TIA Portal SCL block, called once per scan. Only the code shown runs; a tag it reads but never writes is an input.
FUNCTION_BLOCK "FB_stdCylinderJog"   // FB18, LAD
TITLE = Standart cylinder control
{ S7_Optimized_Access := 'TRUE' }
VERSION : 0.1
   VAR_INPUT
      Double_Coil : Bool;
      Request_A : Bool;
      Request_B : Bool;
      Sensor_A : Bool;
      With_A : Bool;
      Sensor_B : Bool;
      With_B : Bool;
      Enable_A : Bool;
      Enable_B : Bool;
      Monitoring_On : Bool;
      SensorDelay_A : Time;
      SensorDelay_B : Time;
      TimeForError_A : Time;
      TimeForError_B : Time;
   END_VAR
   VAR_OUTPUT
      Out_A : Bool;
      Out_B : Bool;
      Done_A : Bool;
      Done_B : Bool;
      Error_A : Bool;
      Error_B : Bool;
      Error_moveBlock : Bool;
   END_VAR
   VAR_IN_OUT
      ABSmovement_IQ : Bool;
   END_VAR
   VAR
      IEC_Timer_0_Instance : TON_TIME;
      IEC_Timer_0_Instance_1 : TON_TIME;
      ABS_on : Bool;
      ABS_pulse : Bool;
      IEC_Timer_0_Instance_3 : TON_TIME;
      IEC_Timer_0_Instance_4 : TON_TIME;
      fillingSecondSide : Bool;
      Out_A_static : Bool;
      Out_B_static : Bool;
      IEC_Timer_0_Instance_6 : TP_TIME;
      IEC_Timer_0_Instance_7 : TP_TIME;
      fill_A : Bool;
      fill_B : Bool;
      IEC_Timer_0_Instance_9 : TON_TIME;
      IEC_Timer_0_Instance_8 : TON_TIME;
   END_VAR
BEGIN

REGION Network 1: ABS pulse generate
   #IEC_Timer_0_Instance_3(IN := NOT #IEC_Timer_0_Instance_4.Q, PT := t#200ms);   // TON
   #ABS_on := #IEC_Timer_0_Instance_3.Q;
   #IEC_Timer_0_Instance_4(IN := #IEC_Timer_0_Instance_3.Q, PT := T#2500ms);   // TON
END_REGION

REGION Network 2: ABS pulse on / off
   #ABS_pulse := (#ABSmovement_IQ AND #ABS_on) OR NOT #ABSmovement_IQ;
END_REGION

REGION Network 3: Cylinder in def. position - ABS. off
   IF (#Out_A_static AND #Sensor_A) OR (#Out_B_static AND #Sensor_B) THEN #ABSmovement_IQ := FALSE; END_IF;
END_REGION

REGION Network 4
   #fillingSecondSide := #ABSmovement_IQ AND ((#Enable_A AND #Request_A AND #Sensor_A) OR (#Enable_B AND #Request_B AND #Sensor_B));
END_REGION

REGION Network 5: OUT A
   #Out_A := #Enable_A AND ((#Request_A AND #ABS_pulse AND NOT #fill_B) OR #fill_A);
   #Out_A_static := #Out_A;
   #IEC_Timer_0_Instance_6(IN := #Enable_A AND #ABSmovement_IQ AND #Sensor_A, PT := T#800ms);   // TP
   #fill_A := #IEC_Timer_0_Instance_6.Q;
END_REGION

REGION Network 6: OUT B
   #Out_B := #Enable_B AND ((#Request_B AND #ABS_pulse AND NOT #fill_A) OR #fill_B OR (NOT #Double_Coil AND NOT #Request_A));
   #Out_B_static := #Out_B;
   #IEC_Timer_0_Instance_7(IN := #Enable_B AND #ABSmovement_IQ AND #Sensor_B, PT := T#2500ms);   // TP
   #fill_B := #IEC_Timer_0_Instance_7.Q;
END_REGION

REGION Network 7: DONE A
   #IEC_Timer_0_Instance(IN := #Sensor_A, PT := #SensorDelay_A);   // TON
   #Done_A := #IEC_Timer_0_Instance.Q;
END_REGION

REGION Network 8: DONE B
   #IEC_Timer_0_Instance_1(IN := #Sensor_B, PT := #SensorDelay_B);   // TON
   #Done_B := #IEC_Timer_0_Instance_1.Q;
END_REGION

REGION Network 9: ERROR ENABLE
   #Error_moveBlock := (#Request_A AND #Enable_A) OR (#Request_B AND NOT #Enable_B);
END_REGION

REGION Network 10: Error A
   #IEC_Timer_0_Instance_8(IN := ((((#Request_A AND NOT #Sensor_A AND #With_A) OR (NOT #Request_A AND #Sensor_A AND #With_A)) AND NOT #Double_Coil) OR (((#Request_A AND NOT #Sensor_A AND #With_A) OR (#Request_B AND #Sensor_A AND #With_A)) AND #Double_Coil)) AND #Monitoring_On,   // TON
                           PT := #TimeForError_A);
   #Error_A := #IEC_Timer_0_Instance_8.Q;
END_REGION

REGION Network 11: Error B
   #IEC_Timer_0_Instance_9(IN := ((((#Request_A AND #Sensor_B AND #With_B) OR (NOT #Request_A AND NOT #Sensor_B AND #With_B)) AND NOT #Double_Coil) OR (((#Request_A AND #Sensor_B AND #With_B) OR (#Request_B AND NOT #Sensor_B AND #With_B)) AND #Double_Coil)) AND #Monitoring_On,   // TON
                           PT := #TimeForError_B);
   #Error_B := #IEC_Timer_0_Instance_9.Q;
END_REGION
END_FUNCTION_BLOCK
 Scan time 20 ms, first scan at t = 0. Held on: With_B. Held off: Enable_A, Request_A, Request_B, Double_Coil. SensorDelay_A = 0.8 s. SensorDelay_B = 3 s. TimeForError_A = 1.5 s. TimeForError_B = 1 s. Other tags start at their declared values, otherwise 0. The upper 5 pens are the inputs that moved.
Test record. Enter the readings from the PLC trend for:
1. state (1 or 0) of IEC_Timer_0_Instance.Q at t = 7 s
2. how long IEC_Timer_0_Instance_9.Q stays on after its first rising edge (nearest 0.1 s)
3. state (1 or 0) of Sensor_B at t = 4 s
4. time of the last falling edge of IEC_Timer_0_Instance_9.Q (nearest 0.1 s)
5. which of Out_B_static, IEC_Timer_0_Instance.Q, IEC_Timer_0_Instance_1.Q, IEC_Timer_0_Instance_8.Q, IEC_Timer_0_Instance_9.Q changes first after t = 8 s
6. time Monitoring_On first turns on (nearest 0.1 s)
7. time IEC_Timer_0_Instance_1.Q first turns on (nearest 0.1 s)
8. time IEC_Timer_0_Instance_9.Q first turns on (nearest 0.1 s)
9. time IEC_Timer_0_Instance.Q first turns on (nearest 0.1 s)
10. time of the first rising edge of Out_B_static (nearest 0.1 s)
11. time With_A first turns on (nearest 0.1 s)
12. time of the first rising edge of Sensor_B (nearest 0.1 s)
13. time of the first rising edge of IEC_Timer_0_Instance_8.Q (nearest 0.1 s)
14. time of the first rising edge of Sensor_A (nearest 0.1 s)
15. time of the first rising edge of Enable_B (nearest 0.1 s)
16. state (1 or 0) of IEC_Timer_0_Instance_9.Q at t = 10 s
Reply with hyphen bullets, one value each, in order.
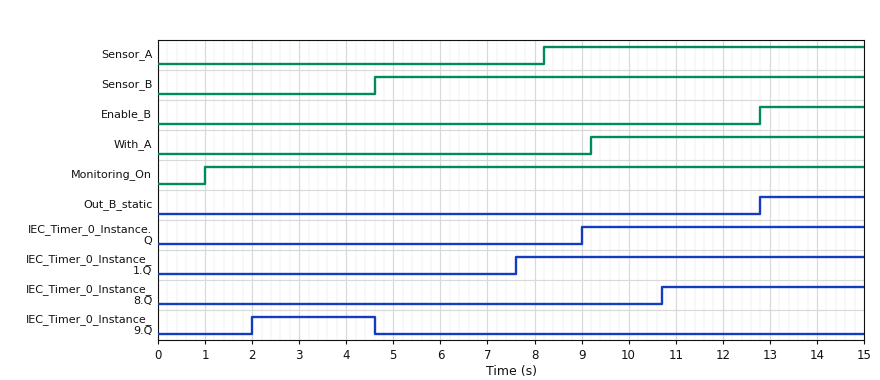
- 0
- 2.6 s
- 0
- 4.6 s
- IEC_Timer_0_Instance.Q
- 1.0 s
- 7.6 s
- 2.0 s
- 9.0 s
- 12.8 s
- 9.2 s
- 4.6 s
- 10.7 s
- 8.2 s
- 12.8 s
- 0
